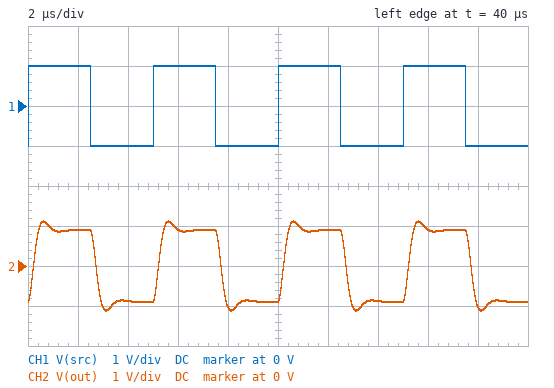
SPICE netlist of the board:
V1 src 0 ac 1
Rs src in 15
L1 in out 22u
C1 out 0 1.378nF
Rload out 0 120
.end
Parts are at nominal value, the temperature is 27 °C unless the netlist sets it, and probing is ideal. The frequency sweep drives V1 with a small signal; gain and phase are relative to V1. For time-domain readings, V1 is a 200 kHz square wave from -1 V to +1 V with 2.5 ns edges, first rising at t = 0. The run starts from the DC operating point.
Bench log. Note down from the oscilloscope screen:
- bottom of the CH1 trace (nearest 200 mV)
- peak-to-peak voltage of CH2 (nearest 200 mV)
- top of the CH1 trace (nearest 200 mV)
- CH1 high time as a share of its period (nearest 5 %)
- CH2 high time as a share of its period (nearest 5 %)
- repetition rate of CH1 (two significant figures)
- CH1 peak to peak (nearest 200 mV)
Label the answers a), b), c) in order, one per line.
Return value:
a) -1.0 V
b) 2.2 V
c) 1.0 V
d) 50 %
e) 50 %
f) 200 kHz
g) 2.0 V
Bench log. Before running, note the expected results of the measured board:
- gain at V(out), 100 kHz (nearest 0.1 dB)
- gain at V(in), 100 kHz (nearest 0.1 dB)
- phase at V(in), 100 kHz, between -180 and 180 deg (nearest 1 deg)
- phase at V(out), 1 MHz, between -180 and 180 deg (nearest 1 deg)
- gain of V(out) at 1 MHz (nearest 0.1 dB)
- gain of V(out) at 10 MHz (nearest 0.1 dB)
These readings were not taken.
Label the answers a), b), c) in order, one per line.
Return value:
a) -1.0 dB
b) -1.0 dB
c) 0 deg
d) -93 deg
e) -2.2 dB
f) -41.5 dB
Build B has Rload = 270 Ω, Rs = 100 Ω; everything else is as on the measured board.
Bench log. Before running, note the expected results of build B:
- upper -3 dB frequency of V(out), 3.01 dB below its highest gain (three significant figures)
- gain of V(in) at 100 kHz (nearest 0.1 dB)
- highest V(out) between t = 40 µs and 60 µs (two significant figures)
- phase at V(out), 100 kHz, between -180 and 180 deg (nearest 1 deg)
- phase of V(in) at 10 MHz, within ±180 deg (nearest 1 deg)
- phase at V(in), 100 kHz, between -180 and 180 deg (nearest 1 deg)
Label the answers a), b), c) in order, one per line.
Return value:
a) 1.23 MHz
b) -2.8 dB
c) 930 mV
d) -6 deg
e) 4 deg
f) -3 deg
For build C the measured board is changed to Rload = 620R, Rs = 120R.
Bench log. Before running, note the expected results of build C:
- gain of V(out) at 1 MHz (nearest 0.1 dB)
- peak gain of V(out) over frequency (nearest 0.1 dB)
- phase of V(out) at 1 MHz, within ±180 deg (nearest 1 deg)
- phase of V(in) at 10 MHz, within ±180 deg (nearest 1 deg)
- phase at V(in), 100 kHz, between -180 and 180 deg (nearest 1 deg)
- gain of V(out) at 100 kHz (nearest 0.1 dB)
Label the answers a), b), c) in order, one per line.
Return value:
a) -2.0 dB
b) -0.6 dB
c) -90 deg
d) 5 deg
e) -5 deg
f) -1.5 dB
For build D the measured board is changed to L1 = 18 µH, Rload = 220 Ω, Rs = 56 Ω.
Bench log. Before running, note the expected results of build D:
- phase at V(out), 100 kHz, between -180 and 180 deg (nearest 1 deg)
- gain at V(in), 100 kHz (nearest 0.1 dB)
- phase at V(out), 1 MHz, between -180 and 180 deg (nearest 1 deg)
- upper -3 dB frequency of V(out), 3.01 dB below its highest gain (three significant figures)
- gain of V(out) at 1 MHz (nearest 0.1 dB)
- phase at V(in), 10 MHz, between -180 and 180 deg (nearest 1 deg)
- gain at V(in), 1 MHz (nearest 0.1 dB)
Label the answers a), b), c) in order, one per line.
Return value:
a) -5 deg
b) -2.0 dB
c) -75 deg
d) 1.34 MHz
e) -0.3 dB
f) 3 deg
g) -6.1 dB
